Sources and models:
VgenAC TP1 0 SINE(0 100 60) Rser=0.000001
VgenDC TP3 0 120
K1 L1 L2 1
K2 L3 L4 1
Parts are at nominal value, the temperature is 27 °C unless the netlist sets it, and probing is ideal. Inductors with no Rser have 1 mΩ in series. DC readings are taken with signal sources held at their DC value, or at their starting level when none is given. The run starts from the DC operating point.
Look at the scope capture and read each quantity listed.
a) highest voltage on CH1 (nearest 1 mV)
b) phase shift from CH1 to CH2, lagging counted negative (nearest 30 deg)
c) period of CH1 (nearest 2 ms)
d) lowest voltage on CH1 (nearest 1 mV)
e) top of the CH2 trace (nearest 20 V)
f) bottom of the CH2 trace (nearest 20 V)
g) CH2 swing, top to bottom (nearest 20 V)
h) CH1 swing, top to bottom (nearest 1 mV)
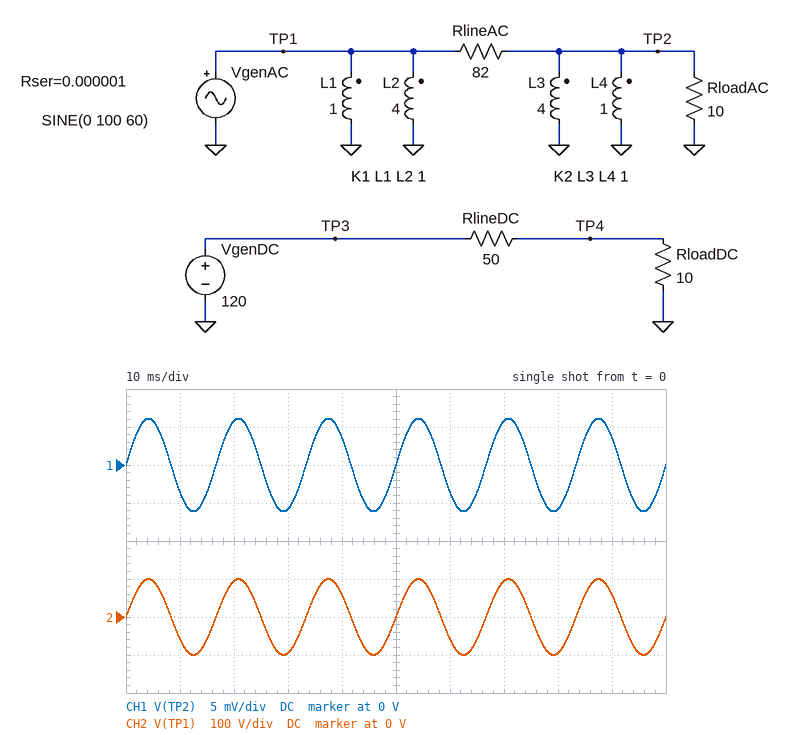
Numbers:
6 mV
0 deg
16 ms
-6 mV
100 V
-100 V
200 V
12 mV
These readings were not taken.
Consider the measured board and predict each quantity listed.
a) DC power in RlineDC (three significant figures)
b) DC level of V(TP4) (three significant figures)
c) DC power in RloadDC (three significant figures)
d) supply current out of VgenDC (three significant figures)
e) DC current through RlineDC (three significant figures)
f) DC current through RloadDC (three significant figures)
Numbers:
200 W
20.0 V
40.0 W
2.00 A
2.00 A
2.00 A
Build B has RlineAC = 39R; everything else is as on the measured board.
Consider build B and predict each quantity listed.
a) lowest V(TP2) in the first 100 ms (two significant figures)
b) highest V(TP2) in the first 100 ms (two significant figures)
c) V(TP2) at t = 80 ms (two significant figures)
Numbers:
-13 mV
13 mV
-12 mV
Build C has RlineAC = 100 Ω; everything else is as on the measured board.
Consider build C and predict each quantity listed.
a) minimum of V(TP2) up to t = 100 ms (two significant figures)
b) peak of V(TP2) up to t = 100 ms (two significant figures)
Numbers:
-5.0 mV
5.0 mV
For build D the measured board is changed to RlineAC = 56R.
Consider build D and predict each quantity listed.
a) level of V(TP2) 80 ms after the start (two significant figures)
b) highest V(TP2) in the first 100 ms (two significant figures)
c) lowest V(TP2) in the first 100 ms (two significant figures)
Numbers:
-8.5 mV
8.9 mV
-8.9 mV
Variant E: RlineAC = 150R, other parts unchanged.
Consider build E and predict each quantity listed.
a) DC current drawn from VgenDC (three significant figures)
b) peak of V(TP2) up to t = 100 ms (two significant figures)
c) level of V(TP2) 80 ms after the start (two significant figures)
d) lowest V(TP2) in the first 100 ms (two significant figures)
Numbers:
2.00 A
3.3 mV
-3.2 mV
-3.3 mV
